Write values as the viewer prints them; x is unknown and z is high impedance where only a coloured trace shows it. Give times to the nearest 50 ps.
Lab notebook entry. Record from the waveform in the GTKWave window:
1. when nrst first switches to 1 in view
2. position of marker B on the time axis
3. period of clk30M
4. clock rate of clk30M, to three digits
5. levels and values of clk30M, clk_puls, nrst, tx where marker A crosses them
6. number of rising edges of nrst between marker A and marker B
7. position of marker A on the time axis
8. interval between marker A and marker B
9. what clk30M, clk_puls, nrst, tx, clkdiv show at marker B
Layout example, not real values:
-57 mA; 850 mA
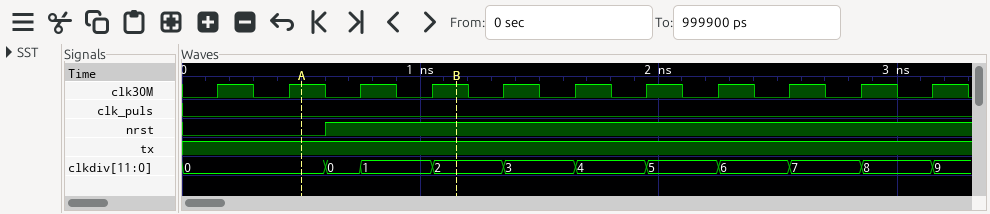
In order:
600 ps; 1150 ps; 300 ps; 3.33 GHz; clk30M=1, clk_puls=0, nrst=0, tx=1; 1; 500 ps; 650 ps; clk30M=1, clk_puls=0, nrst=1, tx=1, clkdiv=2
